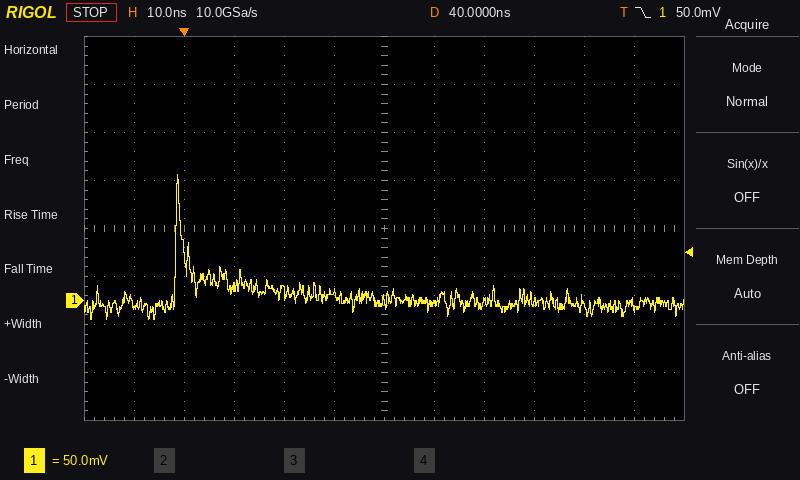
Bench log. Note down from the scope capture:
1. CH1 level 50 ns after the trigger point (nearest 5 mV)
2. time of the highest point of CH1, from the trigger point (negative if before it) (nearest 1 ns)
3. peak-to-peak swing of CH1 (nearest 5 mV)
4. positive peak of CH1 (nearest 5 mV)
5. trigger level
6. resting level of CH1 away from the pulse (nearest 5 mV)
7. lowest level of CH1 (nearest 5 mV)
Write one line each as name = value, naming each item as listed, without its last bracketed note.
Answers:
CH1 level 50 ns after the trigger point = -5 mV
time of the highest point of CH1, from the trigger point (negative if before it) = -1 ns
peak-to-peak swing of CH1 = 150 mV
positive peak of CH1 = 130 mV
trigger level = 50.0 mV
resting level of CH1 away from the pulse = 0 mV
lowest level of CH1 = -20 mV
